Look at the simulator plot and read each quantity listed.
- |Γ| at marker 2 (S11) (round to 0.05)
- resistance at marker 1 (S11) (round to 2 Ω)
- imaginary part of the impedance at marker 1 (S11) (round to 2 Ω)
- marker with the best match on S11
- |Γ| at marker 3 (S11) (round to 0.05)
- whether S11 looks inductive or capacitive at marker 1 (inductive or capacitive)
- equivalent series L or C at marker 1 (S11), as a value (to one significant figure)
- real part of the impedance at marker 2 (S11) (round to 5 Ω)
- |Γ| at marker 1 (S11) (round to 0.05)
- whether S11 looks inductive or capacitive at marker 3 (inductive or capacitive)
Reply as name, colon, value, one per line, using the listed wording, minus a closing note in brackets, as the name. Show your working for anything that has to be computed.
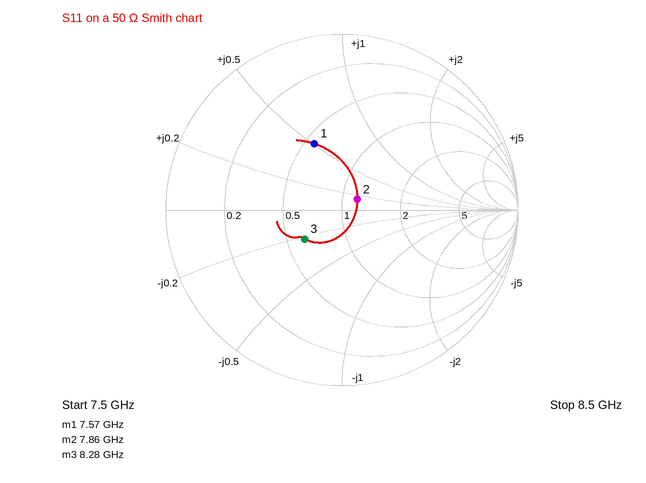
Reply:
|Γ| at marker 2 (S11): 0.10
resistance at marker 1 (S11): 28 Ω
imaginary part of the impedance at marker 1 (S11): +26 Ω
marker with the best match on S11: marker 2
|Γ| at marker 3 (S11): 0.25
whether S11 looks inductive or capacitive at marker 1: inductive
equivalent series L or C at marker 1 (S11), as a value: L = 26 Ω/(2π × 7.57 GHz) ≈ 547 pH, so 500 pH to one significant figure
real part of the impedance at marker 2 (S11): 60 Ω
|Γ| at marker 1 (S11): 0.40
whether S11 looks inductive or capacitive at marker 3: capacitive
